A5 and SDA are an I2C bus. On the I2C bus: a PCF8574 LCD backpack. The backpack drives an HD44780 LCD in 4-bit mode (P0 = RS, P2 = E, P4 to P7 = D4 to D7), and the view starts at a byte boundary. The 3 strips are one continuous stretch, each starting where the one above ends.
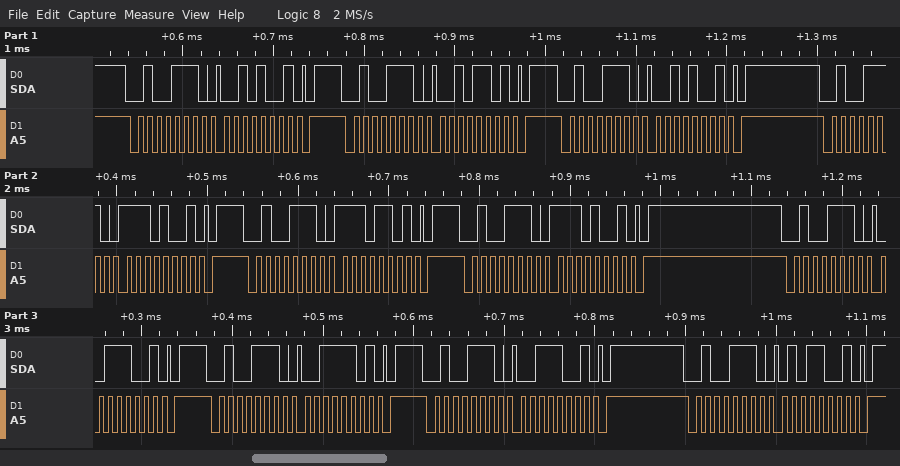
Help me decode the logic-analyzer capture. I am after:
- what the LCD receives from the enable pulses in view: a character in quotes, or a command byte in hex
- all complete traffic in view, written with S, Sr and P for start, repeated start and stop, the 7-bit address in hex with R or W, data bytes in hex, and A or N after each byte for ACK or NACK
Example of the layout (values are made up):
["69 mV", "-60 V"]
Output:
["'.'", "S 27W A 29 A P S 27W A 2D A P S 27W A 29 A P S 27W A E9 A P S 27W A ED A P S 27W A E9 A P S 27W A 39 A P S 27W A 3D A P S 27W A 39 A P S 27W A 59 A P"]
